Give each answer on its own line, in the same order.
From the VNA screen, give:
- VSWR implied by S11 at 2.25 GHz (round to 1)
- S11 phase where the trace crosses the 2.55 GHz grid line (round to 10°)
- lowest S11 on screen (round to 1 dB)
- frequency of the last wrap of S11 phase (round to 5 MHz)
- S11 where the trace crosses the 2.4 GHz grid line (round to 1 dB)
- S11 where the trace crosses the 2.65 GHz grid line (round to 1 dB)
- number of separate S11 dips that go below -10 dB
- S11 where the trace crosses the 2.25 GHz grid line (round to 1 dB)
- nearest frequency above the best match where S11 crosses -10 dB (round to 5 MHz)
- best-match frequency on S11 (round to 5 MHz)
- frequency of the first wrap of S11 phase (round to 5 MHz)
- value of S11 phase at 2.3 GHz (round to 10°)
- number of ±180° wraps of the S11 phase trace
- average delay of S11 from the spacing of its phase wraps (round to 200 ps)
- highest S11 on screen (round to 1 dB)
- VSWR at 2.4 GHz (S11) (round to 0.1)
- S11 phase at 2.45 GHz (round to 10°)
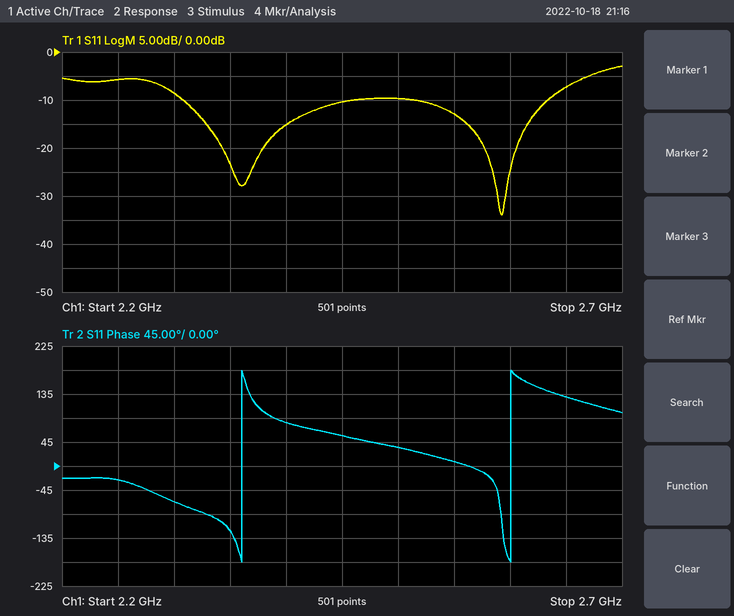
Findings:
3
10°
-34 dB
2.600 GHz
-15 dB
-7 dB
2
-6 dB
2.635 GHz
2.590 GHz
2.360 GHz
-70°
2
4.2 ns
-3 dB
1.4
60°
